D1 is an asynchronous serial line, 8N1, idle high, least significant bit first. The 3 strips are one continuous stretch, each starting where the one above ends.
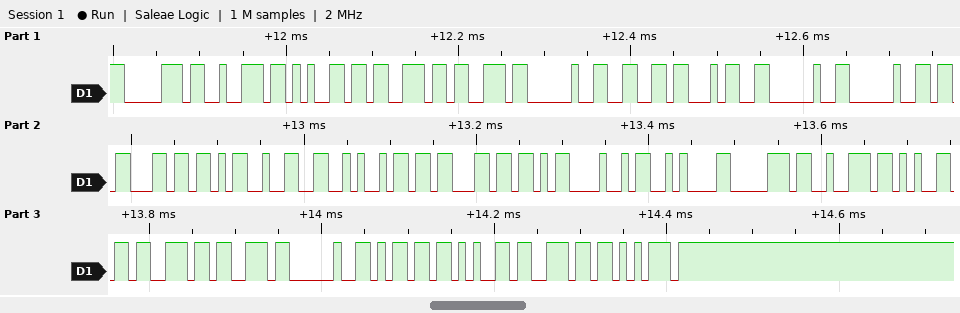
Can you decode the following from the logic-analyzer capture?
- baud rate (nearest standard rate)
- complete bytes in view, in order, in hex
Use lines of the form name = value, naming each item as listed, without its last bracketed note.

baud rate = 115200 baud
complete bytes in view, in order, in hex = 70 72 65 73 73 20 66 34 20 20 1B 5B 32 4A 1B 5B 48 0A 70 72 65 73 73 20 6D 65 6E 75
